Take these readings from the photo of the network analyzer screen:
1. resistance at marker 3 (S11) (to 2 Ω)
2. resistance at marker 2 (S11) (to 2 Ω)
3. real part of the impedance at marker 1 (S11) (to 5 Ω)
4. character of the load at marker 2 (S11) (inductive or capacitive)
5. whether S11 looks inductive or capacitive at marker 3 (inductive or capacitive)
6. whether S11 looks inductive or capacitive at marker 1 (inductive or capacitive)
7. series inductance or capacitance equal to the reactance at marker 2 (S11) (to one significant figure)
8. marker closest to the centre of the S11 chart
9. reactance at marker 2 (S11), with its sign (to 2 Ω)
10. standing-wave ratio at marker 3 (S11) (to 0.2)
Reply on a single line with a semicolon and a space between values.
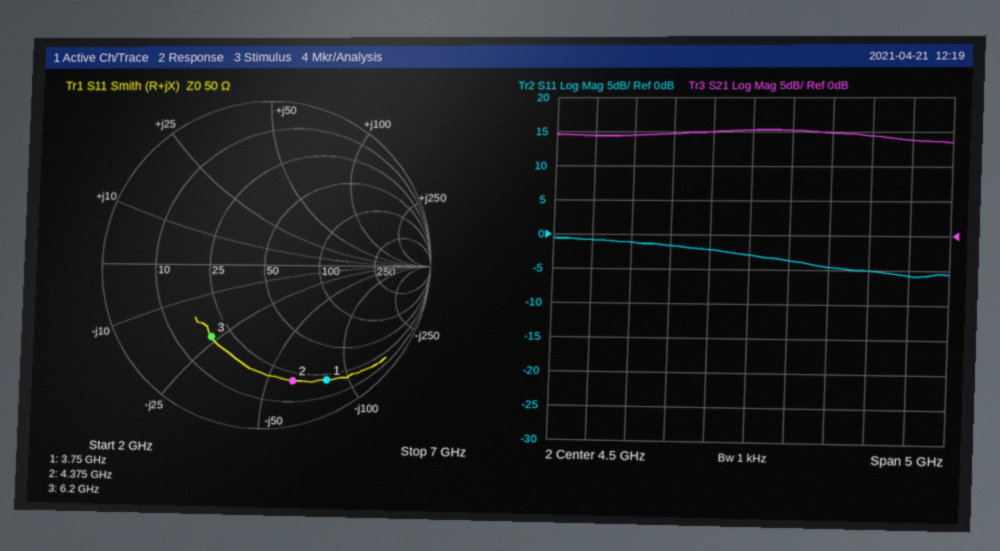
18 Ω; 20 Ω; 20 Ω; capacitive; capacitive; capacitive; 600 fF; marker 3; -62 Ω; 3.4
